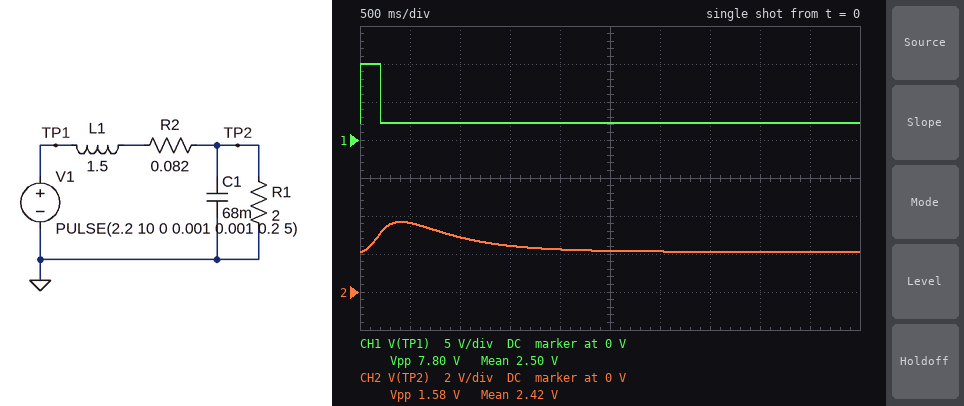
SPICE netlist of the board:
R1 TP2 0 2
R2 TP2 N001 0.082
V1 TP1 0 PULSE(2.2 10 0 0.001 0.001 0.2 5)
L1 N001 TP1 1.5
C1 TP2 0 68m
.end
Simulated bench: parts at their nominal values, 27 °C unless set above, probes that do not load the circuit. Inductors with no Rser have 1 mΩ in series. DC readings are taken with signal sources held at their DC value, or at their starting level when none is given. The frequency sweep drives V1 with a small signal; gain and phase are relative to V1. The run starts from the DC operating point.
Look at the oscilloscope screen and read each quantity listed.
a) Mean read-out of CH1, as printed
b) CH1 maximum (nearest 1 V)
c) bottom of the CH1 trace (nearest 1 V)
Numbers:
2.50 V
10 V
2 V
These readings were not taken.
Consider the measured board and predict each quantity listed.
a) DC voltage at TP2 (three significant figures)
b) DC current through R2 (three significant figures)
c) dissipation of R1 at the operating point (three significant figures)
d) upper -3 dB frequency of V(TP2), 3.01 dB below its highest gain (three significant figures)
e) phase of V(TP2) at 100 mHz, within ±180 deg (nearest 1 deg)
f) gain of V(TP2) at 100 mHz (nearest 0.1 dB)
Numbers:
2.11 V
1.06 A
2.23 W
266 mHz
-25 deg
-0.9 dB
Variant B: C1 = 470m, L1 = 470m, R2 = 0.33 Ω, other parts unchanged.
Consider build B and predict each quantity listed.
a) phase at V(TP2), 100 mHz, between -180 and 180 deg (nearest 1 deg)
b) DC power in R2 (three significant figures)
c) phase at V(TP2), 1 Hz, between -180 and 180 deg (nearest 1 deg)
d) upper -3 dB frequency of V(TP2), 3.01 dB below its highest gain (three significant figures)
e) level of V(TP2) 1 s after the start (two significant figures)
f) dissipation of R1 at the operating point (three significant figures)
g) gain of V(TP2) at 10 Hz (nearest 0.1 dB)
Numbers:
-13 deg
294 mW
-162 deg
435 mHz
3.3 V
1.78 W
-58.8 dB
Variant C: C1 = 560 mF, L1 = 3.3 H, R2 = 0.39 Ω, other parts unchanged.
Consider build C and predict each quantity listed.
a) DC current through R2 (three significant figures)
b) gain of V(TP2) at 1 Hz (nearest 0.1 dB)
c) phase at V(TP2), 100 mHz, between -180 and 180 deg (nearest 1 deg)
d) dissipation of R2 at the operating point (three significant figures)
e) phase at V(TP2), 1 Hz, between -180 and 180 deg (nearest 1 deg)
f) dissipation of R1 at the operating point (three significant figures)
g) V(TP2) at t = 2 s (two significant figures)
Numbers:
920 mA
-37.2 dB
-68 deg
330 mW
-171 deg
1.69 W
2.3 V
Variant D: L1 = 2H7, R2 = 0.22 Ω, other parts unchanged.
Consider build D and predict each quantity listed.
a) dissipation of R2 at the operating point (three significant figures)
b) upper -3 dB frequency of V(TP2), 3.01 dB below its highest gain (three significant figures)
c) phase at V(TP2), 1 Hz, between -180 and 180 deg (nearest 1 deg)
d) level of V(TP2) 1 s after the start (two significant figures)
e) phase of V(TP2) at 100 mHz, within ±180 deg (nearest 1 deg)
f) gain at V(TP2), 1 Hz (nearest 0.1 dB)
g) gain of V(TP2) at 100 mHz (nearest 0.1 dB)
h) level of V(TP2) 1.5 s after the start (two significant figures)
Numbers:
216 mW
145 mHz
-126 deg
2.6 V
-40 deg
-20.5 dB
-2.6 dB
2.4 V
